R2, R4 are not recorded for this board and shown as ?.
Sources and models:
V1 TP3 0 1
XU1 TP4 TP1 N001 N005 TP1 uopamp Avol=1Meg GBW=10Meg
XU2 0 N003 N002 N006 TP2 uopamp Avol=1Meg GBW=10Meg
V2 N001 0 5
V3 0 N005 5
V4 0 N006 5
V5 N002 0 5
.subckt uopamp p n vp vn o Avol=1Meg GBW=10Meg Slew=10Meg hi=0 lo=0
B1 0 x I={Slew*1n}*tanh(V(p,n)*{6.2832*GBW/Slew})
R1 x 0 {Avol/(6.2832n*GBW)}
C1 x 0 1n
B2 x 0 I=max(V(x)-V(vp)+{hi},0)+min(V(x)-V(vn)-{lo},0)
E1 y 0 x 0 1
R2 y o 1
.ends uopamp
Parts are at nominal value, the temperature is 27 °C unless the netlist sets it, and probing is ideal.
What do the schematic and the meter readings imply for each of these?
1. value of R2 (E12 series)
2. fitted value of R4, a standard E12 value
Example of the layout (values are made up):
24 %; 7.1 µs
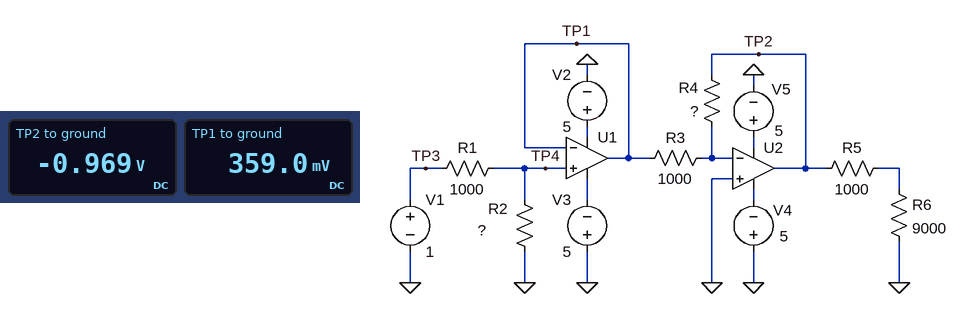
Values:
560 Ω; 2.7 kΩ
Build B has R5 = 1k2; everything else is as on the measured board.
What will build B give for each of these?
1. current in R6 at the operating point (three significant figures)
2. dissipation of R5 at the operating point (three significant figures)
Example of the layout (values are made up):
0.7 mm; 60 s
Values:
95.0 µA; 10.8 µW
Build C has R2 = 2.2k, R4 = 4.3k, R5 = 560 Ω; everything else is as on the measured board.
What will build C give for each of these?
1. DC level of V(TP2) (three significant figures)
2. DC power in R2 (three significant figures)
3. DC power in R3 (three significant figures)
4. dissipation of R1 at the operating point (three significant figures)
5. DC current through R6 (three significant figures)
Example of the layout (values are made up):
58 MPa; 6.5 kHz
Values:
-2.96 V; 215 µW; 473 µW; 97.7 µW; 309 µA
